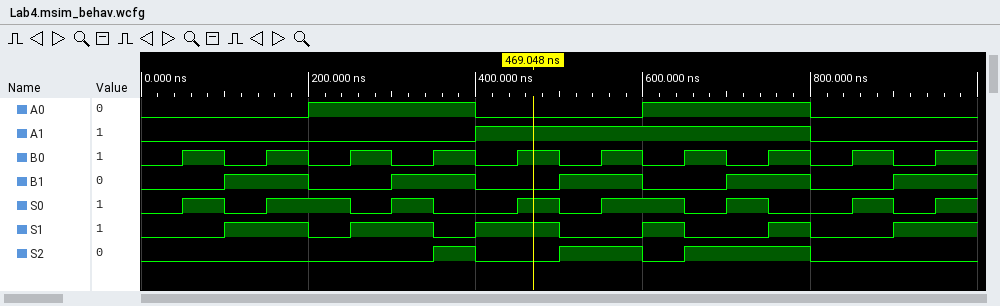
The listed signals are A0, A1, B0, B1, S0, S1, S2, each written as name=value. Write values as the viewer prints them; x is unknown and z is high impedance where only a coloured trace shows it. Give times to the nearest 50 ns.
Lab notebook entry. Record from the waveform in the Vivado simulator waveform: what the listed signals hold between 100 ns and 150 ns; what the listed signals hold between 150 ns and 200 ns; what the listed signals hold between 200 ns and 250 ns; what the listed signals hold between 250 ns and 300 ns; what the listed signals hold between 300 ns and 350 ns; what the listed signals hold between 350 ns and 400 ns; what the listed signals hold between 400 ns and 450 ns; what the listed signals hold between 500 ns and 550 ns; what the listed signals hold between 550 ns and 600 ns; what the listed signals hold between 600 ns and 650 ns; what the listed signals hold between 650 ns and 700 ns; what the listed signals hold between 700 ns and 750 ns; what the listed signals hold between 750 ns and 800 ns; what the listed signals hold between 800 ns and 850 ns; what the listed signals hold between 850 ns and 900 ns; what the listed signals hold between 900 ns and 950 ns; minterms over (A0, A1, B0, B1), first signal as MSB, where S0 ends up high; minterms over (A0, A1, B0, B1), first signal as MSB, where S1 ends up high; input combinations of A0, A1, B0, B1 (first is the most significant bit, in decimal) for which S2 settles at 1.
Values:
A0=0, A1=0, B0=0, B1=1, S0=0, S1=1, S2=0
A0=0, A1=0, B0=1, B1=1, S0=1, S1=1, S2=0
A0=1, A1=0, B0=0, B1=0, S0=1, S1=0, S2=0
A0=1, A1=0, B0=1, B1=0, S0=0, S1=1, S2=0
A0=1, A1=0, B0=0, B1=1, S0=1, S1=1, S2=0
A0=1, A1=0, B0=1, B1=1, S0=0, S1=0, S2=1
A0=0, A1=1, B0=0, B1=0, S0=0, S1=1, S2=0
A0=0, A1=1, B0=0, B1=1, S0=0, S1=0, S2=1
A0=0, A1=1, B0=1, B1=1, S0=1, S1=0, S2=1
A0=1, A1=1, B0=0, B1=0, S0=1, S1=1, S2=0
A0=1, A1=1, B0=1, B1=0, S0=0, S1=0, S2=1
A0=1, A1=1, B0=0, B1=1, S0=1, S1=0, S2=1
A0=1, A1=1, B0=1, B1=1, S0=0, S1=1, S2=1
A0=0, A1=0, B0=0, B1=0, S0=0, S1=0, S2=0
A0=0, A1=0, B0=1, B1=0, S0=1, S1=0, S2=0
A0=0, A1=0, B0=0, B1=1, S0=0, S1=1, S2=0
2, 3, 6, 7, 8, 9, 12, 13
1, 3, 4, 6, 9, 10, 12, 15
5, 7, 11, 13, 14, 15
